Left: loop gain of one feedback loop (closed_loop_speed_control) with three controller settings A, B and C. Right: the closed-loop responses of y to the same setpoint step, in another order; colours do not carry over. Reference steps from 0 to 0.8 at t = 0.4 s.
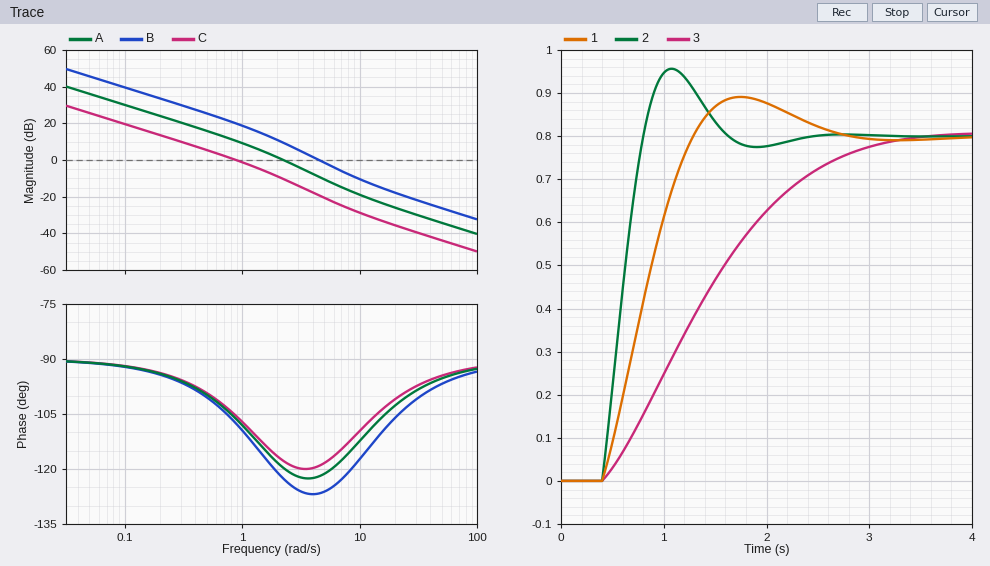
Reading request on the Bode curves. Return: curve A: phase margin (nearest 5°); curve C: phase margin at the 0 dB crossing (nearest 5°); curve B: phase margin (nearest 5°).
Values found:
60°
75°
55°
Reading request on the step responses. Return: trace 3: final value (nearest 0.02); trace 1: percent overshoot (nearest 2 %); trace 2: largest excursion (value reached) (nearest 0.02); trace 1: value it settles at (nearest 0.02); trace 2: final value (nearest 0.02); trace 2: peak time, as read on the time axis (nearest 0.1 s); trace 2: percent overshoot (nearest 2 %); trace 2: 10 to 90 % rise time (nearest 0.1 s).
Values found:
0.80
12 %
0.96
0.80
0.80
1.1 s
20 %
0.3 s
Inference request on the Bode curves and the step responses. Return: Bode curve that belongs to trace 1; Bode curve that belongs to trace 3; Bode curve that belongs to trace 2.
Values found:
A
C
B
